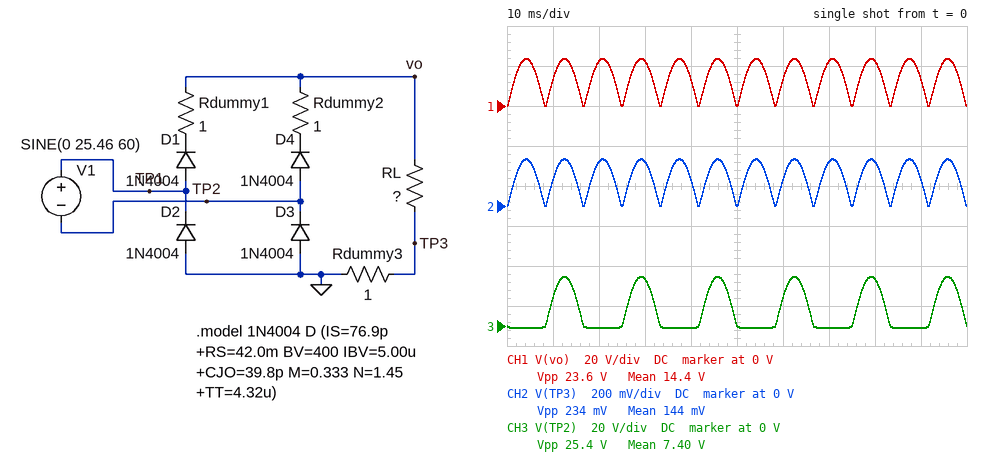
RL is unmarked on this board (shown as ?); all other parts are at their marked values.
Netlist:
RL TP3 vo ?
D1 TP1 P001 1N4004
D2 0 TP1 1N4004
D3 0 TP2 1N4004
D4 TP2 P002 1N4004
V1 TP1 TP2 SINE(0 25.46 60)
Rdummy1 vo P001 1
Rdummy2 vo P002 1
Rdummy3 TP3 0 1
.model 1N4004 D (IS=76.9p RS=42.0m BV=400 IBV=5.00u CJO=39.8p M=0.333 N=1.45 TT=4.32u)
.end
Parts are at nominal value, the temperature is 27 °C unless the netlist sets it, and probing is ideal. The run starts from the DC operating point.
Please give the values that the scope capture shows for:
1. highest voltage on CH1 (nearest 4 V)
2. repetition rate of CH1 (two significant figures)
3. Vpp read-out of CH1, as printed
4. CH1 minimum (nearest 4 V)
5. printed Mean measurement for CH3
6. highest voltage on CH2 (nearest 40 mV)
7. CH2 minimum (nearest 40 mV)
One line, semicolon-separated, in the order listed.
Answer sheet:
24 V; 120 Hz; 23.6 V; 0 V; 7.40 V; 240 mV; 0 V
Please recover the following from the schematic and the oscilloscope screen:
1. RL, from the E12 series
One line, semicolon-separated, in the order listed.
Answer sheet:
100 Ω
